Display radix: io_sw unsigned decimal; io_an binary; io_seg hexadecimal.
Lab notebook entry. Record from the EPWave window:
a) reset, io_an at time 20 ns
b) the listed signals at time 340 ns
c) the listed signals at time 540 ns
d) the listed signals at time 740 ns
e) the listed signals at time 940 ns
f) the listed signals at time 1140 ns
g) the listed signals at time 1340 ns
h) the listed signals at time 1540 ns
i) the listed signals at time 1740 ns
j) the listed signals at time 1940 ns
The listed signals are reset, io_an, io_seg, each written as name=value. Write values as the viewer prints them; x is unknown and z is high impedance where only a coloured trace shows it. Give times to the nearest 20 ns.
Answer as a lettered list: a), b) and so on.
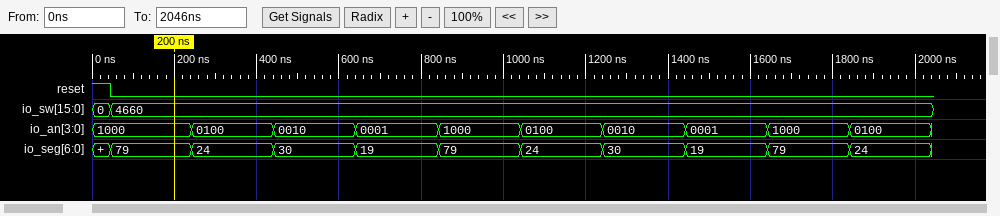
a) reset=1, io_an=1000
b) reset=0, io_an=0100, io_seg=24
c) reset=0, io_an=0010, io_seg=30
d) reset=0, io_an=0001, io_seg=19
e) reset=0, io_an=1000, io_seg=79
f) reset=0, io_an=0100, io_seg=24
g) reset=0, io_an=0010, io_seg=30
h) reset=0, io_an=0001, io_seg=19
i) reset=0, io_an=1000, io_seg=79
j) reset=0, io_an=0100, io_seg=24
